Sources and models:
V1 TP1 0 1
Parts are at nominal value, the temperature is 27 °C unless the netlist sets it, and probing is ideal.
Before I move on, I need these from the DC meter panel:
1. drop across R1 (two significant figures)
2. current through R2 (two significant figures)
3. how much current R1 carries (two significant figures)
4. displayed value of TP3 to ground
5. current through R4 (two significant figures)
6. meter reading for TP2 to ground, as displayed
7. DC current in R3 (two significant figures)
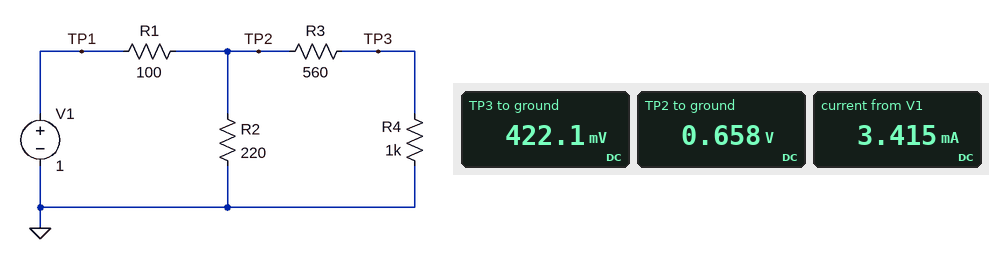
340 mV
3.0 mA
3.4 mA
422.1 mV
420 µA
0.658 V
420 µA
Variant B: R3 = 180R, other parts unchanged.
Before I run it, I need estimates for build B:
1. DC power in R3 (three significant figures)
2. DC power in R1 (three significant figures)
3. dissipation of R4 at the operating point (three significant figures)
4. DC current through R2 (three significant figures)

54.6 µW
1.23 mW
303 µW
2.95 mA
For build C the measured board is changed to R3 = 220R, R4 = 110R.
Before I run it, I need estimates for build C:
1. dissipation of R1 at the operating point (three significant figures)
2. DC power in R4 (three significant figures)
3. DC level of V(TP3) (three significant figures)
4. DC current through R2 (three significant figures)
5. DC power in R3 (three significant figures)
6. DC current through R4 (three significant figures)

1.86 mW
327 µW
190 mV
2.59 mA
654 µW
1.72 mA
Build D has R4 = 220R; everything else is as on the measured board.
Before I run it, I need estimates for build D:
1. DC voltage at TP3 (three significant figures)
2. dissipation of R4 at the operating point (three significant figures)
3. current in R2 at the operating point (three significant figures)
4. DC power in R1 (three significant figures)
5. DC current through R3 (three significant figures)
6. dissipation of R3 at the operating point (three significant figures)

178 mV
144 µW
2.87 mA
1.36 mW
810 µA
367 µW
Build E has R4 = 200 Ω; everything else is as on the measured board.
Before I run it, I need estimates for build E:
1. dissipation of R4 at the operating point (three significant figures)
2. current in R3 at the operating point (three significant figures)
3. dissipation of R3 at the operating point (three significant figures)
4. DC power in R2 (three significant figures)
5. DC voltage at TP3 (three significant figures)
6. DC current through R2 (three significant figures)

138 µW
830 µA
385 µW
1.81 mW
166 mV
2.87 mA
